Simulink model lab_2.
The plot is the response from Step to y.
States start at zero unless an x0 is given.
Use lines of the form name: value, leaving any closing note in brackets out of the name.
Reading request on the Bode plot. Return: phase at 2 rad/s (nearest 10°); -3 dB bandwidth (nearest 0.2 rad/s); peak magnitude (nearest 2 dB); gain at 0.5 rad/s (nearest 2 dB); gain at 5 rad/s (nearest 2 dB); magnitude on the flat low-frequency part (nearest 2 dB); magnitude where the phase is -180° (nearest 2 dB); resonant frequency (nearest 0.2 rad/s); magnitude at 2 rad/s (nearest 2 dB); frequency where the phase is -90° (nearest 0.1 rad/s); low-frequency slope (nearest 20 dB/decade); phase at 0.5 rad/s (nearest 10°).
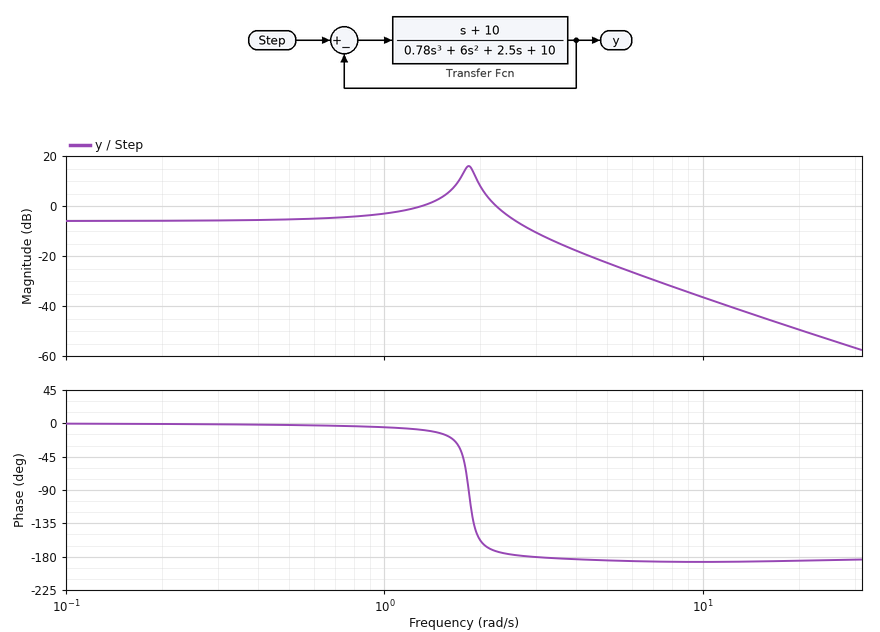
phase at 2 rad/s: -160°
-3 dB bandwidth: 2.8 rad/s
peak magnitude: 16 dB
gain at 0.5 rad/s: -6 dB
gain at 5 rad/s: -22 dB
magnitude on the flat low-frequency part: -6 dB
magnitude where the phase is -180°: -10 dB
resonant frequency: 1.8 rad/s
magnitude at 2 rad/s: 8 dB
frequency where the phase is -90°: 1.8 rad/s
low-frequency slope: 0 dB/decade
phase at 0.5 rad/s: 0°
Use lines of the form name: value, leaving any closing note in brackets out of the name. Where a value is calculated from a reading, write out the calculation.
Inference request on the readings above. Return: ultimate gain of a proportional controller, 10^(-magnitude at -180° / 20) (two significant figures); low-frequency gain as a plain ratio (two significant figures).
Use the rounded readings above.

ultimate gain of a proportional controller, 10^(-magnitude at -180° / 20): 10^(10 / 20) = 3.2
low-frequency gain as a plain ratio: 10^(-6 / 20) = 0.50
